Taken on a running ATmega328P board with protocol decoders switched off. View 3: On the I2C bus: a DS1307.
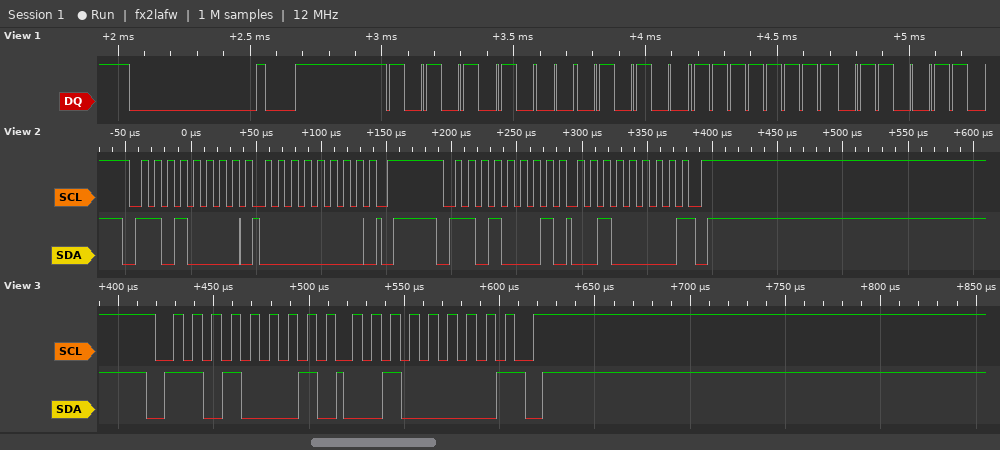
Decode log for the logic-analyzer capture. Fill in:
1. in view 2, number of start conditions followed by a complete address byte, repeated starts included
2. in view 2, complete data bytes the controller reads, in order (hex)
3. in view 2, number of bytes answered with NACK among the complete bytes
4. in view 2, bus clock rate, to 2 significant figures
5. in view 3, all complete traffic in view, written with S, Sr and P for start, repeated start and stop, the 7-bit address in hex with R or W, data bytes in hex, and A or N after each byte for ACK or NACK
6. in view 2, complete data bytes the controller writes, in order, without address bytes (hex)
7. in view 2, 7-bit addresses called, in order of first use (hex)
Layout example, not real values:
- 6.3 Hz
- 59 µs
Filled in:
- 2
- 20
- 1
- 100 kHz
- S 68R A 20 N P
- 00
- 0x68
